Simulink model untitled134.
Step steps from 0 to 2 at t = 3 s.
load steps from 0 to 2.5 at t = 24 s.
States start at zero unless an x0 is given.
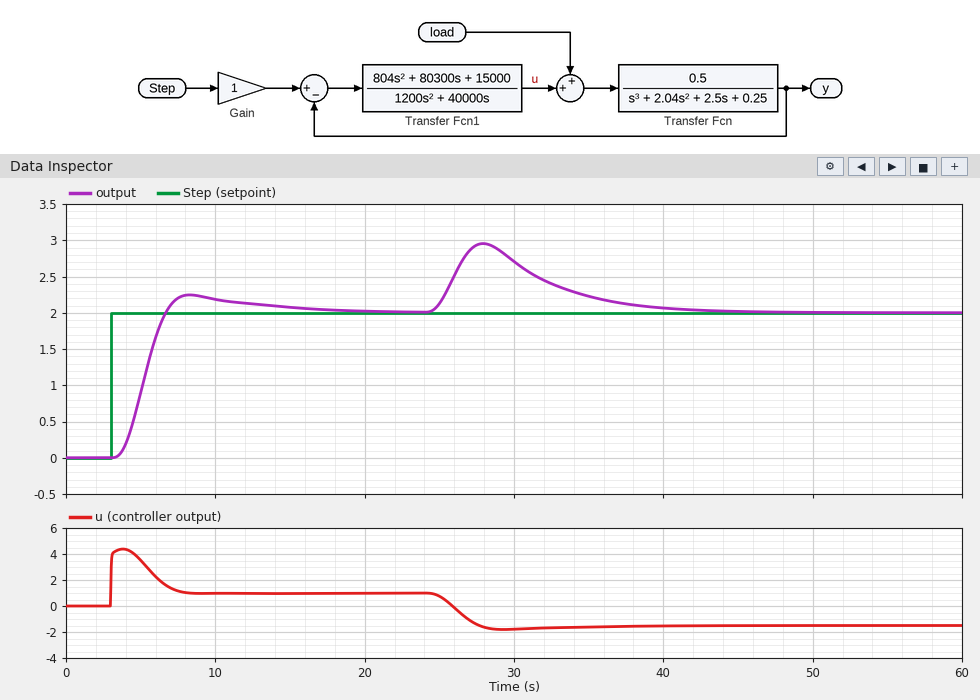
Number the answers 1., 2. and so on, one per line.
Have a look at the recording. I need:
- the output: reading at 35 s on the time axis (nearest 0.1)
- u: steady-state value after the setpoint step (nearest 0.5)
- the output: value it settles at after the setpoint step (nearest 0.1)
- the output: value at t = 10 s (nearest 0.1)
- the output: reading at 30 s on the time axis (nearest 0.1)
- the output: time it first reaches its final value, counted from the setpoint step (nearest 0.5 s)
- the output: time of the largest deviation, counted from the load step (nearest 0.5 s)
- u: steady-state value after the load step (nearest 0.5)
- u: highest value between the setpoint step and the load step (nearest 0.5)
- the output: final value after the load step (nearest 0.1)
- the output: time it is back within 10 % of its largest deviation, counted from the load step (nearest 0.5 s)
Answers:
1. 2.2
2. 1.0
3. 2.0
4. 2.2
5. 2.7
6. 3.5 s
7. 4.0 s
8. -1.5
9. 4.5
10. 2.0
11. 14.5 s
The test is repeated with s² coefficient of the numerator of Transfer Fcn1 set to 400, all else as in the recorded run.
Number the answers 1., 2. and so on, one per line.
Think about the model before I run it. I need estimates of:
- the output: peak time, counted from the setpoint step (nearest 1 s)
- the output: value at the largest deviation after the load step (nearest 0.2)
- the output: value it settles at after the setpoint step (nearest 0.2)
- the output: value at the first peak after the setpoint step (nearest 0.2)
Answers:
1. 5 s
2. 3.0
3. 2.0
4. 2.2
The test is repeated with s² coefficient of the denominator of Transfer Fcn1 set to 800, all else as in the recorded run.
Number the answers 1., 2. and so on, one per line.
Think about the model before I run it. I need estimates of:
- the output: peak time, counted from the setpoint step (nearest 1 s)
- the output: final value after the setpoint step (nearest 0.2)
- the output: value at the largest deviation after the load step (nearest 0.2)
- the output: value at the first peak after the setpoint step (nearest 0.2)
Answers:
1. 5 s
2. 2.0
3. 3.0
4. 2.2
